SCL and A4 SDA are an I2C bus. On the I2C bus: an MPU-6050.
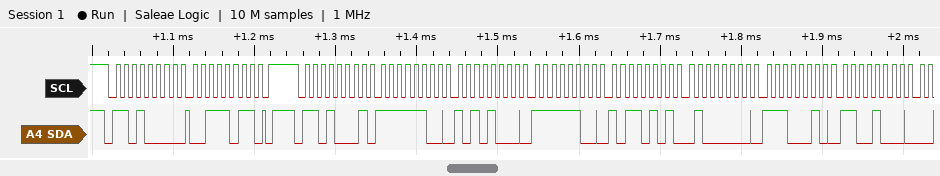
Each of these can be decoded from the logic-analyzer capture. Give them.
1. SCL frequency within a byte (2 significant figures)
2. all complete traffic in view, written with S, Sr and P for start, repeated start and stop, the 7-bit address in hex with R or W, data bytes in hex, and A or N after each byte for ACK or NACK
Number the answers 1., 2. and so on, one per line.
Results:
1. 100 kHz
2. S 68W A 3B A P S 68R A FC A A8 A FC A B5 A 40 A E2 A C8 A
